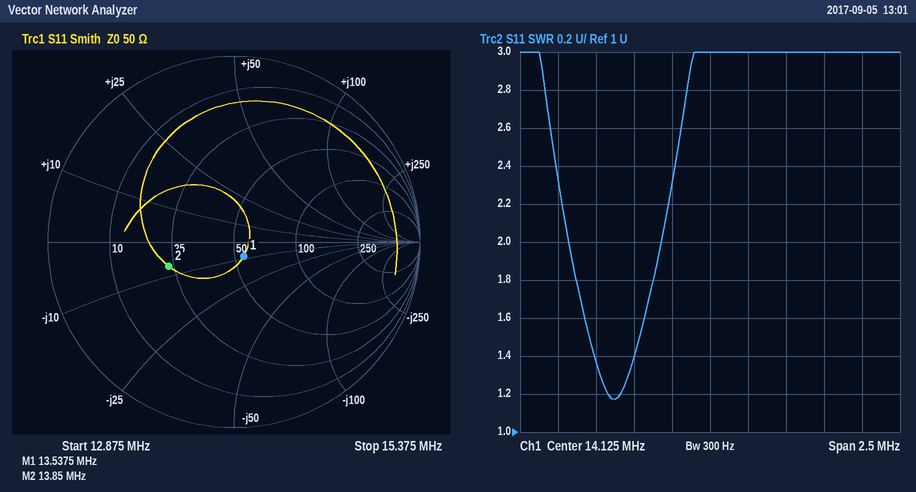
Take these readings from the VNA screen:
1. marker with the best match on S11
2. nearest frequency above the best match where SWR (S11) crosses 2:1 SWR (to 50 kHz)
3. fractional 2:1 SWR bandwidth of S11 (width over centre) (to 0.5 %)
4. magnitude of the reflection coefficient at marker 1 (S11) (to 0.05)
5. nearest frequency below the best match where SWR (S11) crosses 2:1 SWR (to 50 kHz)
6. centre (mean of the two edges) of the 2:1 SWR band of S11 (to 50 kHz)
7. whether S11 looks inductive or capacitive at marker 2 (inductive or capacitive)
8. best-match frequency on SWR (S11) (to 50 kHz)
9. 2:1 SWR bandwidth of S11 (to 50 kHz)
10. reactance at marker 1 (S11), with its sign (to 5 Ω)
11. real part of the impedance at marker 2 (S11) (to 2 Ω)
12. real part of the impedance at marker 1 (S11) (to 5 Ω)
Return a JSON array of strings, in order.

["marker 1", "13.80 MHz", "4.5 %", "0.10", "13.20 MHz", "13.50 MHz", "capacitive", "13.50 MHz", "600 kHz", "-10 Ω", "24 Ω", "55 Ω"]
